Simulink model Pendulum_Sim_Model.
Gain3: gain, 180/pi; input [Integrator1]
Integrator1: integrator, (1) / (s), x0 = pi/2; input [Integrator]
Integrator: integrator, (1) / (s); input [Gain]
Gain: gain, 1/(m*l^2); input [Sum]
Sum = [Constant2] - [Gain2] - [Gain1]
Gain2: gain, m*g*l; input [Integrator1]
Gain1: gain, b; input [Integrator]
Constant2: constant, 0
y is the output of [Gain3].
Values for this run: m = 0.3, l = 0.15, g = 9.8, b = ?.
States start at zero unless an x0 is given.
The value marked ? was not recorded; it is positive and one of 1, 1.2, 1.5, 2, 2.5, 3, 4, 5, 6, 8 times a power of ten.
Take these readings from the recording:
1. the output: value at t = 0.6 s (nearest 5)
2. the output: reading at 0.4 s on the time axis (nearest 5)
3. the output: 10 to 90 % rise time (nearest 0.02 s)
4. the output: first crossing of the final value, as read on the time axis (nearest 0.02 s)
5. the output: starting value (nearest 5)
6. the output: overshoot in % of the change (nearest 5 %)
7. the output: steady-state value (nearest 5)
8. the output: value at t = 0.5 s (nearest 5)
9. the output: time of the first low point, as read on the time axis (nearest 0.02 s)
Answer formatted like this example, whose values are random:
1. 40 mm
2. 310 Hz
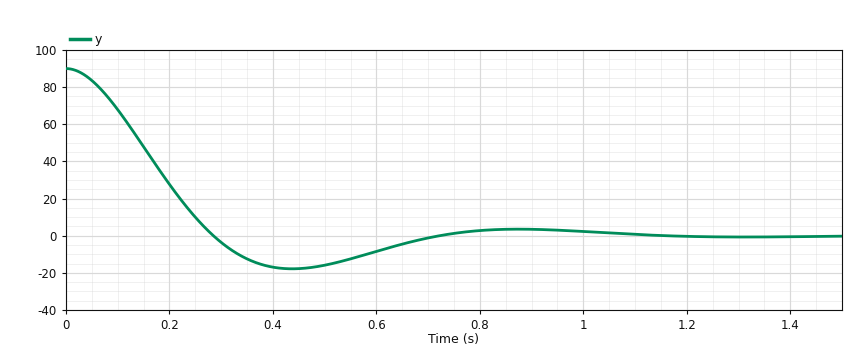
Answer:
1. -10
2. -15
3. 0.20 s
4. 0.28 s
5. 90
6. 20 %
7. 0
8. -15
9. 0.44 s
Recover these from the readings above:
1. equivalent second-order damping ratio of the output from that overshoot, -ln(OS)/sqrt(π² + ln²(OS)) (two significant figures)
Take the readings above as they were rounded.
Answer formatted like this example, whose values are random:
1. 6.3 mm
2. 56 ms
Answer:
1. 0.46
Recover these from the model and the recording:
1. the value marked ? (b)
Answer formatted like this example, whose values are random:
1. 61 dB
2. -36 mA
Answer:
1. 0.05
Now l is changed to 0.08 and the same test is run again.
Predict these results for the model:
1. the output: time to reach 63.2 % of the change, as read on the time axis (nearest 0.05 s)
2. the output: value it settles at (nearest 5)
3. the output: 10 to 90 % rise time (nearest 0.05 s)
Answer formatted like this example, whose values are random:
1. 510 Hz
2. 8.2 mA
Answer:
1. 0.20 s
2. 0
3. 0.40 s
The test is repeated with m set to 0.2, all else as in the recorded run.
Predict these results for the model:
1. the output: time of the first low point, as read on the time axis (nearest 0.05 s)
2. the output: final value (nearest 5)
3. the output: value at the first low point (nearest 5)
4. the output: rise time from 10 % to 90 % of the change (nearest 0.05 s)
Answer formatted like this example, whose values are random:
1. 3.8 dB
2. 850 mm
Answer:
1. 0.55 s
2. 0
3. -5
4. 0.25 s
